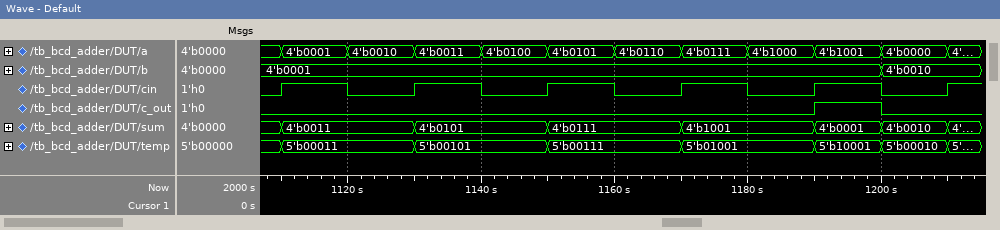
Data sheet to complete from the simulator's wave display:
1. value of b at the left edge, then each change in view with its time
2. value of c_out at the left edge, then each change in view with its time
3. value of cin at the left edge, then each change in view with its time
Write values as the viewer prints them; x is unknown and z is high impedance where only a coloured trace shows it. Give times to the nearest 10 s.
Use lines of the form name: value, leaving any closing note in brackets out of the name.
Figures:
value of b at the left edge, then each change in view with its time: 4'b0001, 4'b0010 at 1200 s
value of c_out at the left edge, then each change in view with its time: 0, 1 at 1190 s, 0 at 1200 s
value of cin at the left edge, then each change in view with its time: 0, 1 at 1110 s, 0 at 1120 s, 1 at 1130 s, 0 at 1140 s, 1 at 1150 s, 0 at 1160 s, 1 at 1170 s, 0 at 1180 s, 1 at 1190 s, 0 at 1200 s, 1 at 1210 s
